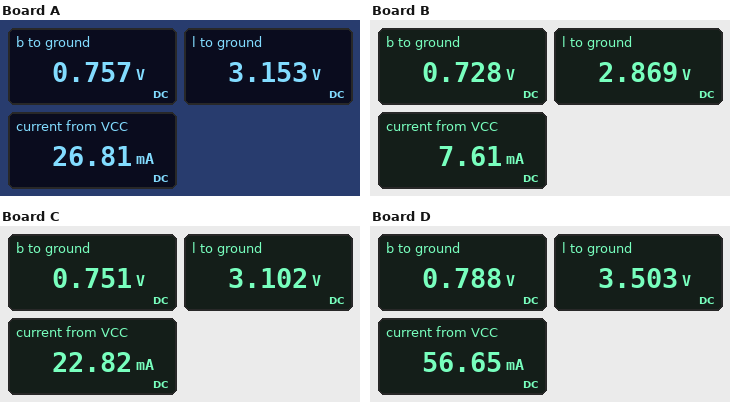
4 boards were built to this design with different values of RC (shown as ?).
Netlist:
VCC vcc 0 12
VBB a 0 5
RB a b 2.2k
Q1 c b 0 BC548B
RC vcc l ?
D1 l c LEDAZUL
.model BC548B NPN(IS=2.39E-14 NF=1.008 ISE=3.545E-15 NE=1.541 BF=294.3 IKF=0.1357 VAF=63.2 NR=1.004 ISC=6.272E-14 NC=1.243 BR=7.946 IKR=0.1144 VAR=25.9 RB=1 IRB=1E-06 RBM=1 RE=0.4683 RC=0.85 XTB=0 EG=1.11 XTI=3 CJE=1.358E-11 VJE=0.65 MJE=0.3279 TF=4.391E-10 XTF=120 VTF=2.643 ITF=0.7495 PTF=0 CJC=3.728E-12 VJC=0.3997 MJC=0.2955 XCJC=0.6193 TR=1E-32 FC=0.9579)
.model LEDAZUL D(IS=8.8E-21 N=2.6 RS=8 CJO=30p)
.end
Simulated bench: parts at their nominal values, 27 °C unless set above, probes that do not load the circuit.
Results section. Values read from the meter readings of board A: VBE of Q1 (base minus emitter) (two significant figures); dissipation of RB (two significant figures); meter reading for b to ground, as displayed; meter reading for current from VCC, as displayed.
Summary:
760 mV
8.2 mW
0.757 V
26.81 mA
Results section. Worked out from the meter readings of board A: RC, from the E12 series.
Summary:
330 Ω
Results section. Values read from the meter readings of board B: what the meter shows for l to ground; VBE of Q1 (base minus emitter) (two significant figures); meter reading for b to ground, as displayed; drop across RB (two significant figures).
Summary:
2.869 V
730 mV
0.728 V
4.3 V
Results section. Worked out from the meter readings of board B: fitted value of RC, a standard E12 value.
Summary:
1.2 kΩ
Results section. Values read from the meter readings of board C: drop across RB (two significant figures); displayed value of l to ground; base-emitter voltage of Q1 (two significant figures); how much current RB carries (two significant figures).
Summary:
4.2 V
3.102 V
750 mV
1.9 mA
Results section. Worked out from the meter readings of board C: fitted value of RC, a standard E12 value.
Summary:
390 Ω
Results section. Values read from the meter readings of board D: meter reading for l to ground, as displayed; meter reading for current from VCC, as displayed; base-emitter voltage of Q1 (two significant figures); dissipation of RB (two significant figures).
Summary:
3.503 V
56.65 mA
790 mV
8.1 mW
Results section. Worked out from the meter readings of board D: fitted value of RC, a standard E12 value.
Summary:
150 Ω
